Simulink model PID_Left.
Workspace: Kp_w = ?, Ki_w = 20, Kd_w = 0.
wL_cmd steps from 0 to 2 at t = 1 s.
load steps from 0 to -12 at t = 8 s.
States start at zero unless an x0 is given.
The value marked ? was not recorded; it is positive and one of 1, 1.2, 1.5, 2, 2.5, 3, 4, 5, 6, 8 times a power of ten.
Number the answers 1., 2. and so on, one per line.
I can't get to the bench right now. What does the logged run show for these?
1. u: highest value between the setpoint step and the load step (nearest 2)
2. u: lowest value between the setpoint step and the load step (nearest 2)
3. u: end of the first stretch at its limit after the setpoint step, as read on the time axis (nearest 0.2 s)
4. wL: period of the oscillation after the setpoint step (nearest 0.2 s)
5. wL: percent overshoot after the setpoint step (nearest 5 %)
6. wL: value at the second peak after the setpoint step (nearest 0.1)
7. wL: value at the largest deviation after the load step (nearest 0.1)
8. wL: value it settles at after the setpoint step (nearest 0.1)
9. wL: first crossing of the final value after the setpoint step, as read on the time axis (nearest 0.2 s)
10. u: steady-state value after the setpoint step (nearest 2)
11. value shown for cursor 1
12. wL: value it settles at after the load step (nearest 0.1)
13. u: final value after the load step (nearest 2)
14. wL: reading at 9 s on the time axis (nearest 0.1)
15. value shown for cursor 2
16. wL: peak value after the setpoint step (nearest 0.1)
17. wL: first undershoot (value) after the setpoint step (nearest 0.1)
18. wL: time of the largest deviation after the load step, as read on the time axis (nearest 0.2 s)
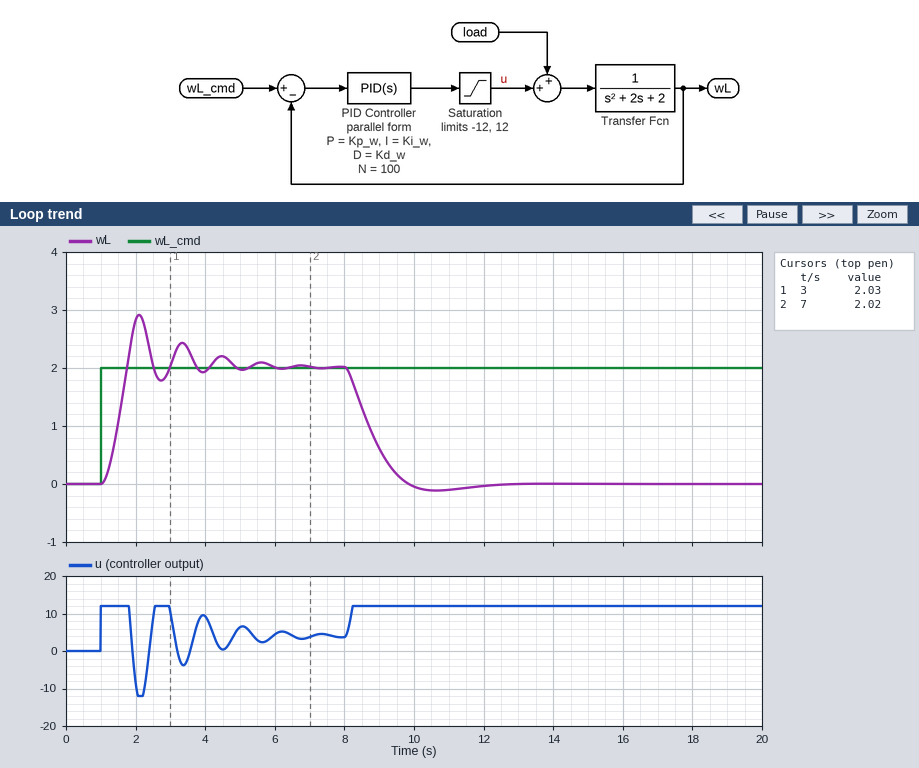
1. 12
2. -12
3. 1.8 s
4. 1.2 s
5. 45 %
6. 2.4
7. -0.1
8. 2.0
9. 1.8 s
10. 4
11. 2.03
12. 0.0
13. 12
14. 0.6
15. 2.02
16. 2.9
17. 1.8
18. 10.6 s
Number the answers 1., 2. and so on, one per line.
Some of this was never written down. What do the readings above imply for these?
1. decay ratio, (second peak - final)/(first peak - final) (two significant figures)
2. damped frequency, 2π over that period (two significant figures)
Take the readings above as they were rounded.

1. 0.44
2. 5.2 rad/s
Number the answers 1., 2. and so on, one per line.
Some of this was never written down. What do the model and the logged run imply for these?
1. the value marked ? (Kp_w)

1. 30
